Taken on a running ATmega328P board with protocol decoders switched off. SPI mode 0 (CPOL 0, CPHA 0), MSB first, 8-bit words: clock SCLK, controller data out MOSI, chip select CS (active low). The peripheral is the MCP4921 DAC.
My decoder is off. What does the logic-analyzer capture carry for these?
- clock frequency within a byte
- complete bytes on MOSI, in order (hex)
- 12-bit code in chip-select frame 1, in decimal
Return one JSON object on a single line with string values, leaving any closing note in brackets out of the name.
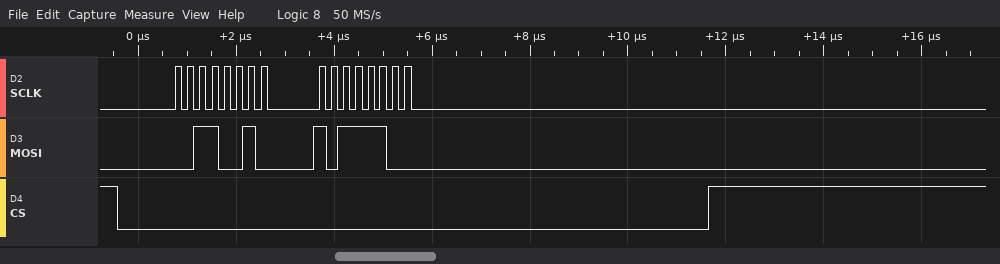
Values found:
{"clock frequency within a byte": "4 MHz", "complete bytes on MOSI, in order": "0x32 0xBC", "12-bit code in chip-select frame 1, in decimal": "700"}
